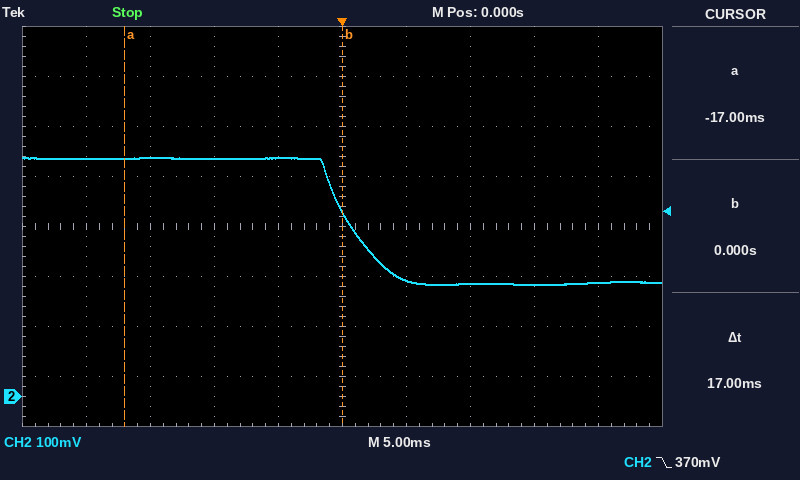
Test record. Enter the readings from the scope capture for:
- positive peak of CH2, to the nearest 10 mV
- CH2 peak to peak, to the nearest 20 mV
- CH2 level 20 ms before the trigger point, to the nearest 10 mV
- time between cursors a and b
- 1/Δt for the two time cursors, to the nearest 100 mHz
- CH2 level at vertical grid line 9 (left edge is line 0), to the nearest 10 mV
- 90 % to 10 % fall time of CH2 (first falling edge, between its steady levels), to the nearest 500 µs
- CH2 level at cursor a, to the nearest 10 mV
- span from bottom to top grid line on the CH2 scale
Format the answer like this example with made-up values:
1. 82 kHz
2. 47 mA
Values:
1. 480 mV
2. 260 mV
3. 480 mV
4. 17 ms
5. 58.8 Hz
6. 230 mV
7. 5.0 ms
8. 480 mV
9. 800 mV
